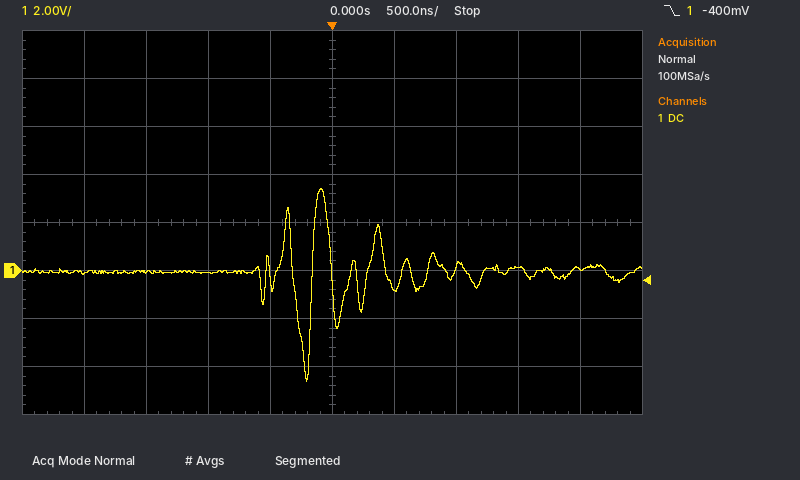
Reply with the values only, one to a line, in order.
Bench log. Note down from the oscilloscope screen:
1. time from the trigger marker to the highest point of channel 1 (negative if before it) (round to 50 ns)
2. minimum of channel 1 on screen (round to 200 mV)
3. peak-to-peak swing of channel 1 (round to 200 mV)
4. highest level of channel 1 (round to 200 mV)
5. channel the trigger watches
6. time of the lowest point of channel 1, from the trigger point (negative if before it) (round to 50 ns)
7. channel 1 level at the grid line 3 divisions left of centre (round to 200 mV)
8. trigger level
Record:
-100 ns
-4.6 V
8.0 V
3.4 V
channel 1
-200 ns
0.0 V
-400 mV
